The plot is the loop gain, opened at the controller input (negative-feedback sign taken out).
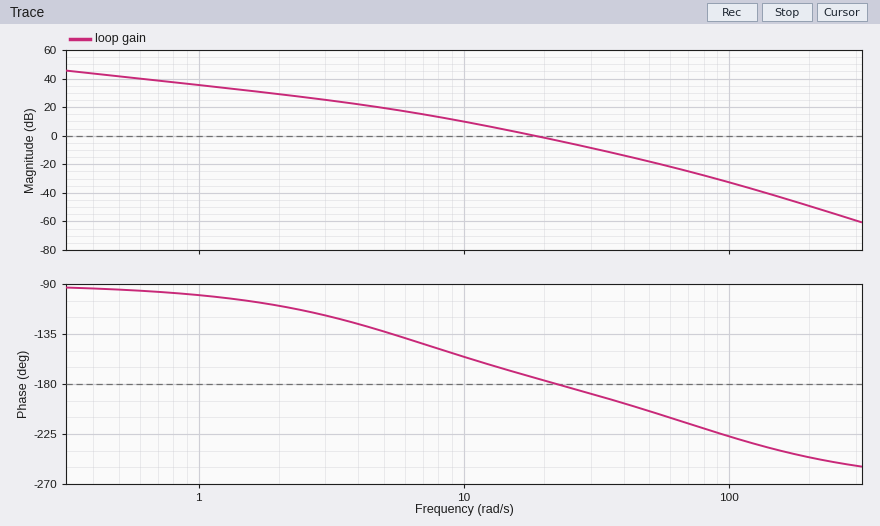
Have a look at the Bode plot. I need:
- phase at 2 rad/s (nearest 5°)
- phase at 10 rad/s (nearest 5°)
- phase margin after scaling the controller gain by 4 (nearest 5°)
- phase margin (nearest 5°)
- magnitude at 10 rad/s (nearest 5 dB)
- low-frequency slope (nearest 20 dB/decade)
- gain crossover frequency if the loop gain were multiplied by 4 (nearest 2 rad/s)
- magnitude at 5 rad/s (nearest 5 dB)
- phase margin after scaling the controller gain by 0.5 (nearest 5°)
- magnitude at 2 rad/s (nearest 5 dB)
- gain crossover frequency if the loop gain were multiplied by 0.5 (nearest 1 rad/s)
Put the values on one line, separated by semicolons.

-110°; -155°; -15°; 5°; 10 dB; -20 dB/decade; 36 rad/s; 20 dB; 15°; 30 dB; 13 rad/s
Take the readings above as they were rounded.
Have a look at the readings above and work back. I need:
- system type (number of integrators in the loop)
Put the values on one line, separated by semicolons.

1
